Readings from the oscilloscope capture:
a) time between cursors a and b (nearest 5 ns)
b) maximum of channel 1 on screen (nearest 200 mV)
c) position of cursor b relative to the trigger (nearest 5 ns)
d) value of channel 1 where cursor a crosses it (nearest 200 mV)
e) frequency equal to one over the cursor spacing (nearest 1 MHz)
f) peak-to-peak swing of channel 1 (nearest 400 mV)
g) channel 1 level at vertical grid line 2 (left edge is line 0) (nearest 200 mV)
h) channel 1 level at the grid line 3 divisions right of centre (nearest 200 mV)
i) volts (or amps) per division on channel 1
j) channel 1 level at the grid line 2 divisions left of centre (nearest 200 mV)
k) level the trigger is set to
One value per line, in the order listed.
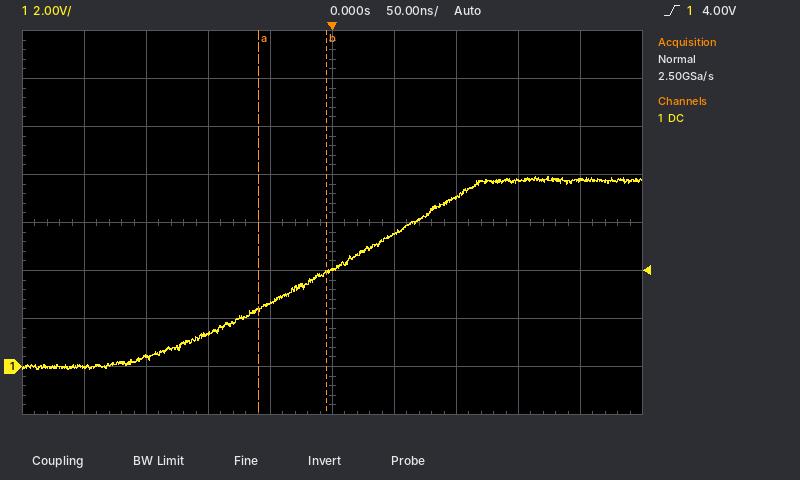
55 ns
8.0 V
-5 ns
2.4 V
18 MHz
8.0 V
400 mV
7.8 V
2 V
1.4 V
4.00 V
